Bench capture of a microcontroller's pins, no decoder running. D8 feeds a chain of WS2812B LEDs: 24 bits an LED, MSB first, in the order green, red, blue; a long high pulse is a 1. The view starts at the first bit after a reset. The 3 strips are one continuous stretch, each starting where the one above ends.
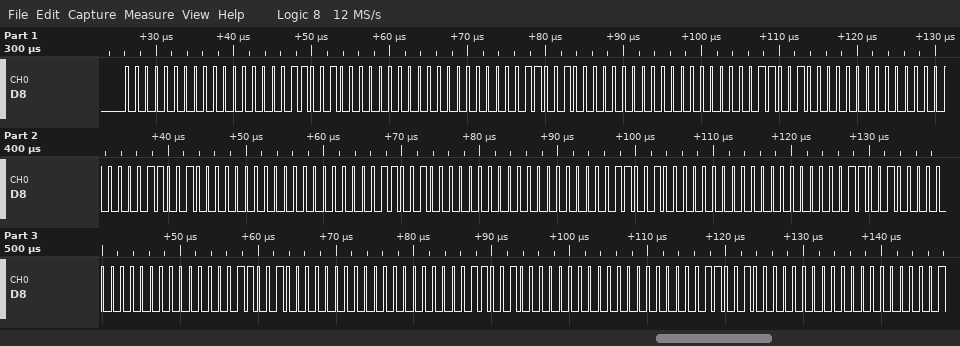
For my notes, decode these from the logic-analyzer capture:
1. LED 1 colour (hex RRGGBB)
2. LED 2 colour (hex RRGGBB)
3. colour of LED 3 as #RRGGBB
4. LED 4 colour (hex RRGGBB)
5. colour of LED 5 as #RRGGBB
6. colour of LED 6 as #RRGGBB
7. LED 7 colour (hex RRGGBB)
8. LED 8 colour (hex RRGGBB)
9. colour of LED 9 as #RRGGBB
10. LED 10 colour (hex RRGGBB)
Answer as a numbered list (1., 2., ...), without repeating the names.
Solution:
1. #000064
2. #000064
3. #000064
4. #000064
5. #000064
6. #000064
7. #000064
8. #000064
9. #000064
10. #000064
